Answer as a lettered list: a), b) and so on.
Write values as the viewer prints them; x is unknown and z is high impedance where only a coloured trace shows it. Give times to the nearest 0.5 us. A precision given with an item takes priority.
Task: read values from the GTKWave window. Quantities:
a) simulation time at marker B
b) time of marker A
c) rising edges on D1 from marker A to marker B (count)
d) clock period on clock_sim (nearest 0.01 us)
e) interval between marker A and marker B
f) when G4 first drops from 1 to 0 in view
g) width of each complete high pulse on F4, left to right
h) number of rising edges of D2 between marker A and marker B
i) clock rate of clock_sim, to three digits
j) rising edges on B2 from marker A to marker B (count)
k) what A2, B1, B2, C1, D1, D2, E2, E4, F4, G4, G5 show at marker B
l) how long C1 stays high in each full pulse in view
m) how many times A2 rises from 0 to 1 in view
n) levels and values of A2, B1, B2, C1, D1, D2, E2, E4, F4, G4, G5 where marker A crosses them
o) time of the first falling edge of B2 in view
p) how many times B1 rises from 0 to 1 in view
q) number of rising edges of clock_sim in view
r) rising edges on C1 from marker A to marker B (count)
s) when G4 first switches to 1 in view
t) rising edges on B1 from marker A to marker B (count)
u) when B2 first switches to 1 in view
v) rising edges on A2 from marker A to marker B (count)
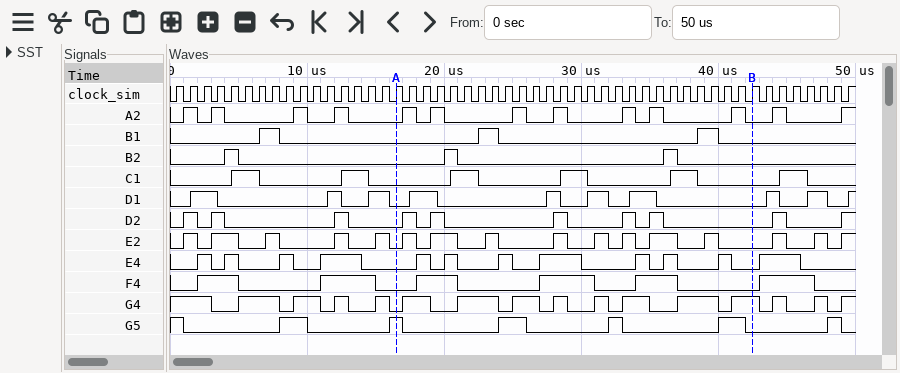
a) 42.5 us
b) 16.5 us
c) 4
d) 1 us
e) 26 us
f) 3 us
g) 3 us, 4 us, 3 us, 4 us, 3 us, 4 us
h) 5
i) 1.00 MHz
j) 2
k) A2=0, B1=0, B2=0, C1=0, D1=0, D2=0, E2=0, E4=0, F4=0, G4=1, G5=0
l) 2 us, 2 us, 2 us, 2 us, 2 us, 2 us
m) 13
n) A2=0, B1=0, B2=0, C1=0, D1=0, D2=0, E2=0, E4=0, F4=0, G4=0, G5=1
o) 5 us
p) 3
q) 50
r) 3
s) 5 us
t) 2
u) 4 us
v) 7
